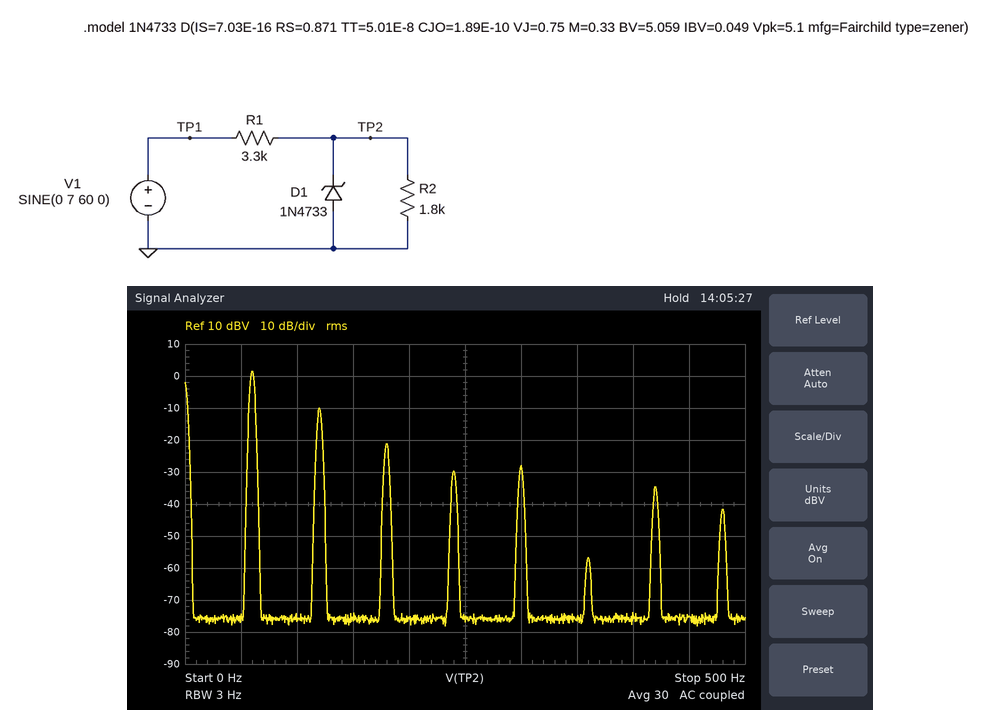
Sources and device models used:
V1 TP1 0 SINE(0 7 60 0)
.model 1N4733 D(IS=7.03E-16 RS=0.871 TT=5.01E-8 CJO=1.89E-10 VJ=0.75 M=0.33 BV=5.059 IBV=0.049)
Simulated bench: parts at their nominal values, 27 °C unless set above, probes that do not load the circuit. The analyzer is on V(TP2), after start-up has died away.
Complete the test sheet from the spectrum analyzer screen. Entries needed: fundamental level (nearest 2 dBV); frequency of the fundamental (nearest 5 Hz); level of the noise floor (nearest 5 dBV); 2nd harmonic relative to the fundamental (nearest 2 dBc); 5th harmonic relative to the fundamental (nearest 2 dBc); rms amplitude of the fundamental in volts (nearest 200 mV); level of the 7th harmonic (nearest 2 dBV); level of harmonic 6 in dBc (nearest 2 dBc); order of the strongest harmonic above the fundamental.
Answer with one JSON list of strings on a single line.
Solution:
["2 dBV", "60 Hz", "-75 dBV", "-12 dBc", "-30 dBc", "1.2 V", "-34 dBV", "-58 dBc", "2"]
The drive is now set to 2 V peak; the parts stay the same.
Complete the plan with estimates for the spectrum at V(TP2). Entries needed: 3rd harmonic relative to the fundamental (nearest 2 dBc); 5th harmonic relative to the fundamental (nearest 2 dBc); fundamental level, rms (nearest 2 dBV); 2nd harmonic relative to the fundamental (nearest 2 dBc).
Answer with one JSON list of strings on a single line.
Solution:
["-36 dBc", "-42 dBc", "-6 dBV", "-36 dBc"]
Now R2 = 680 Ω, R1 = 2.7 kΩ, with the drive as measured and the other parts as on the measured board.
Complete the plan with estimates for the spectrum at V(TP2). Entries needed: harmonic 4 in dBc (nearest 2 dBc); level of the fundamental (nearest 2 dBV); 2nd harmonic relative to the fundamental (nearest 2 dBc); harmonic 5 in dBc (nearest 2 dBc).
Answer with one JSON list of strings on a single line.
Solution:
["-38 dBc", "-2 dBV", "-16 dBc", "-36 dBc"]
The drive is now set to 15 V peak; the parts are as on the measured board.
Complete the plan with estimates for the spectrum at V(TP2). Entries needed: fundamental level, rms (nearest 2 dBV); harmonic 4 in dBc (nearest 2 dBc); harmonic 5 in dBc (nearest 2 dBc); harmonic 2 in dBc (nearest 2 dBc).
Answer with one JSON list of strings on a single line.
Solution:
["6 dBV", "-22 dBc", "-38 dBc", "-10 dBc"]
